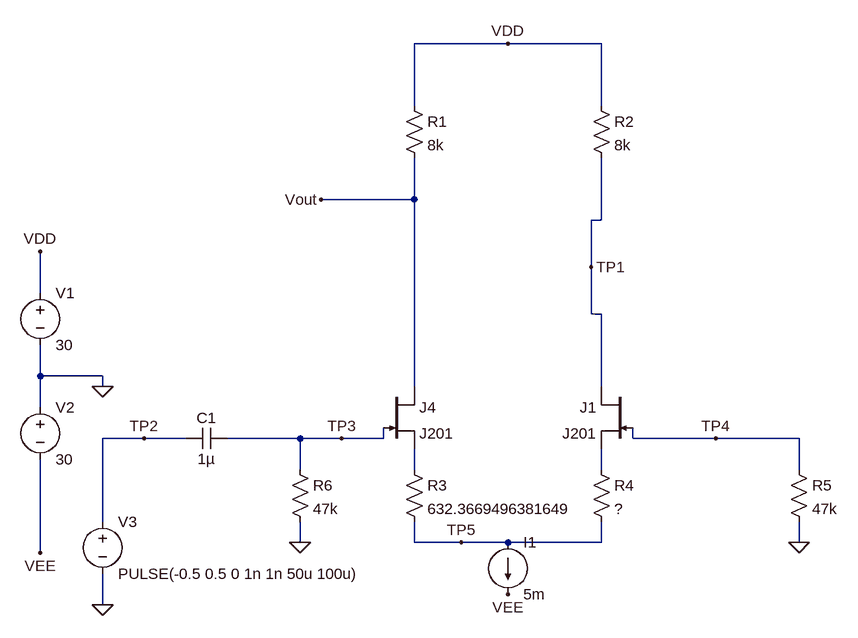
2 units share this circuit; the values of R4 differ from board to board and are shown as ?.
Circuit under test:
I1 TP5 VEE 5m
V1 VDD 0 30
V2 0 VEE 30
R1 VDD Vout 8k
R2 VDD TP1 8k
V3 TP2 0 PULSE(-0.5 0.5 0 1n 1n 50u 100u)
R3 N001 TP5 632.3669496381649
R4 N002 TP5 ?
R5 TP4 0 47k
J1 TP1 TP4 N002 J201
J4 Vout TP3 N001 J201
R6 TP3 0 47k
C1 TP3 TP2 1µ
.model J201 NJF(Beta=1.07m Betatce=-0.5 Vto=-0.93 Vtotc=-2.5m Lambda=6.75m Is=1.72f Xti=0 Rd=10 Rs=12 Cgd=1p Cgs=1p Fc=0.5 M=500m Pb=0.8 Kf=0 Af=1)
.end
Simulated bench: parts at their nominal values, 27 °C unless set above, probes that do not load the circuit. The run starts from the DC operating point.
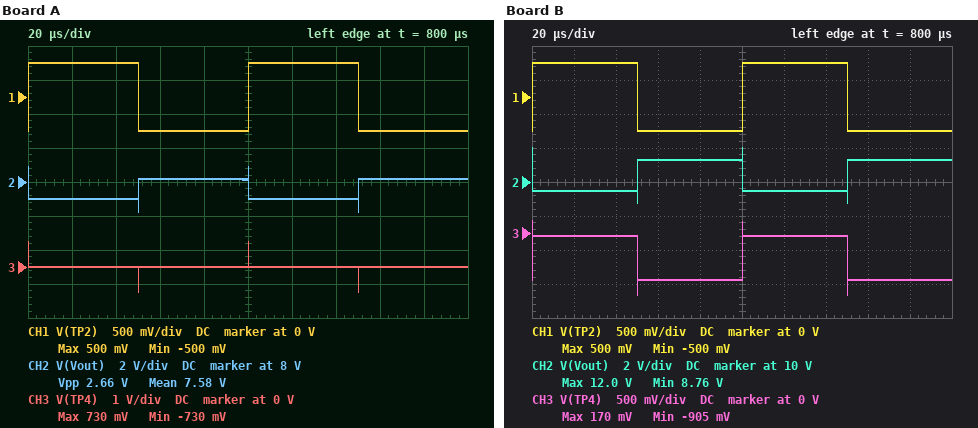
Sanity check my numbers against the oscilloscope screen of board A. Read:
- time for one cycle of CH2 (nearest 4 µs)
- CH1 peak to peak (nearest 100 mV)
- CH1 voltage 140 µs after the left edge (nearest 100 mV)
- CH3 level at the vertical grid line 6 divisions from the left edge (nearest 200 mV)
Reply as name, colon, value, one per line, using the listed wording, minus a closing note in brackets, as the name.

time for one cycle of CH2: 100 µs
CH1 peak to peak: 1.0 V
CH1 voltage 140 µs after the left edge: 500 mV
CH3 level at the vertical grid line 6 divisions from the left edge: 0 V
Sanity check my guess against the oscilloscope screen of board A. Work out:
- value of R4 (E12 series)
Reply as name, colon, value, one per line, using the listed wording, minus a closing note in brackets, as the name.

value of R4: 1.8 kΩ
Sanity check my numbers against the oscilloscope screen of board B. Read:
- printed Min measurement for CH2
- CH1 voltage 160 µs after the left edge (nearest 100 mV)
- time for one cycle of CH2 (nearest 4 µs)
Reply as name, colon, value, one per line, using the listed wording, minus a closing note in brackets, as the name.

printed Min measurement for CH2: 8.76 V
CH1 voltage 160 µs after the left edge: -500 mV
time for one cycle of CH2: 100 µs
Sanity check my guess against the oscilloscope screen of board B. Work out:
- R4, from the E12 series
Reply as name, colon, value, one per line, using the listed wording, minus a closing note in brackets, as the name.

R4, from the E12 series: 270 Ω
